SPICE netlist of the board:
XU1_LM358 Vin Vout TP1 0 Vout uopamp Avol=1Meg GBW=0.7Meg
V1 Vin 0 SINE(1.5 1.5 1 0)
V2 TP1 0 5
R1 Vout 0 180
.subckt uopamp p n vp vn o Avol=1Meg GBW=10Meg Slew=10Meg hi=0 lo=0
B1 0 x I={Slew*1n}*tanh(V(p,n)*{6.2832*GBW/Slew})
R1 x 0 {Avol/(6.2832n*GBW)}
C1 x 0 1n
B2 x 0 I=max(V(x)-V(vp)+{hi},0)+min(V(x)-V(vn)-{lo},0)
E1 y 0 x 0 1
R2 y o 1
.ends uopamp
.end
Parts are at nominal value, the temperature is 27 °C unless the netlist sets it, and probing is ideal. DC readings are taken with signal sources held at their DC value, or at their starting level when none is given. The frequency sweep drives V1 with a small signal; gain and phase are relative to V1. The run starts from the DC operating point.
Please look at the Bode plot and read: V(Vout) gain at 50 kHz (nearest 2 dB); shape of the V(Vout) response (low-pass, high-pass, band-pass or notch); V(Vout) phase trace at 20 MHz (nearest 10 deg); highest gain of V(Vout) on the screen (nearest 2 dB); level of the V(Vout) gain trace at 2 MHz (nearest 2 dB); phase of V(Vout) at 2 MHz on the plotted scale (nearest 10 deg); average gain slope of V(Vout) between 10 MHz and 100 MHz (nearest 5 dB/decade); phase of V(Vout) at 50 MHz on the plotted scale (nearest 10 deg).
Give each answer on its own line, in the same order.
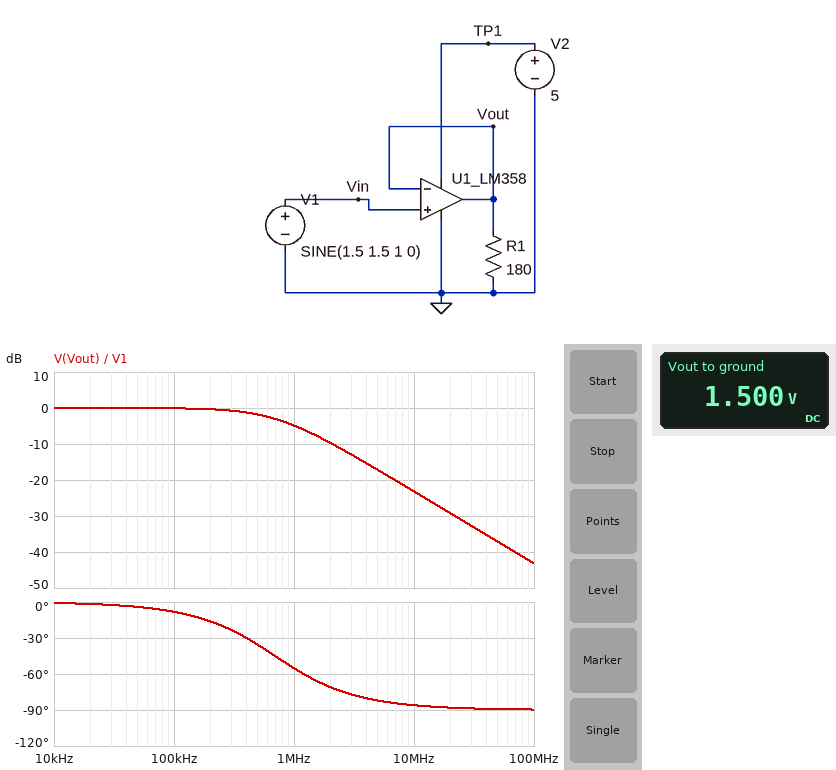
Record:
0 dB
low-pass
-90 deg
0 dB
-10 dB
-70 deg
-20 dB/decade
-90 deg
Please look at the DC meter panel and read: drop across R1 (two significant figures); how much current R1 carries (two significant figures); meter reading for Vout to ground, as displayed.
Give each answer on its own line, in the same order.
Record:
1.5 V
8.3 mA
1.500 V
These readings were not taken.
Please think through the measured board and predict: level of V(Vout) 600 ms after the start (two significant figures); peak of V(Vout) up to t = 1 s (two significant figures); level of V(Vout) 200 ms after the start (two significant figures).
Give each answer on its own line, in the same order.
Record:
620 mV
3.0 V
2.9 V
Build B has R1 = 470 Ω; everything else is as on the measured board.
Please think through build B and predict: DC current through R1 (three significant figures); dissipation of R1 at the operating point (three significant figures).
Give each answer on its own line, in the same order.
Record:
3.19 mA
4.79 mW
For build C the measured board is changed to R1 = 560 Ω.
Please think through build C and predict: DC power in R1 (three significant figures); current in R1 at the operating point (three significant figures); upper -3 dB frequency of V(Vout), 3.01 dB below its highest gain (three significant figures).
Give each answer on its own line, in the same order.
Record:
4.02 mW
2.68 mA
699 kHz
